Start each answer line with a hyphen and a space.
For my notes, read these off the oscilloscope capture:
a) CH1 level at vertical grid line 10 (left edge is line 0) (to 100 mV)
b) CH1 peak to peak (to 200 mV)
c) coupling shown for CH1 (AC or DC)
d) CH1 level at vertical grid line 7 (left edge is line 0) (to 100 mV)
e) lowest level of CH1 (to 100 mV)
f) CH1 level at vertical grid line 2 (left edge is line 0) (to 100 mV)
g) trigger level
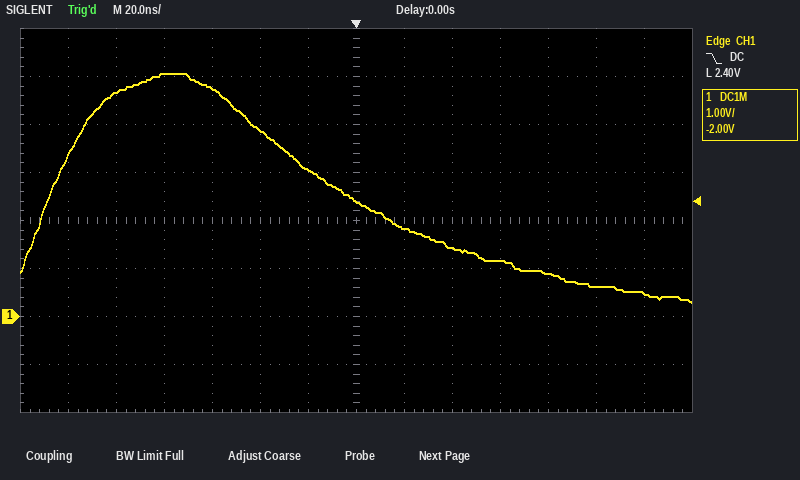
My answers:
- 1.2 V
- 4.8 V
- DC
- 2.4 V
- 300 mV
- 4.7 V
- 2.40 V
